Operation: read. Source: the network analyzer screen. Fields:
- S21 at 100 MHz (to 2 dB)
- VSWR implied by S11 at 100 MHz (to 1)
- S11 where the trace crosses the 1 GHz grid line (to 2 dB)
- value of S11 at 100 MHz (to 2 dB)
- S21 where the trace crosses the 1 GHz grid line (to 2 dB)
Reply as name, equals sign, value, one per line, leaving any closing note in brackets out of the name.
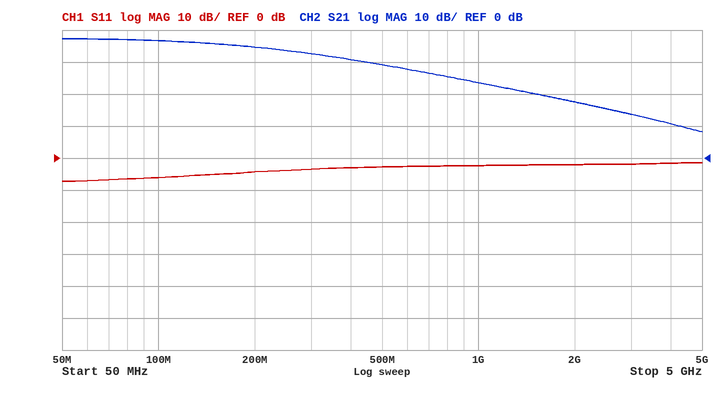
S21 at 100 MHz = 36 dB
VSWR implied by S11 at 100 MHz = 3
S11 where the trace crosses the 1 GHz grid line = -2 dB
value of S11 at 100 MHz = -6 dB
S21 where the trace crosses the 1 GHz grid line = 24 dB
